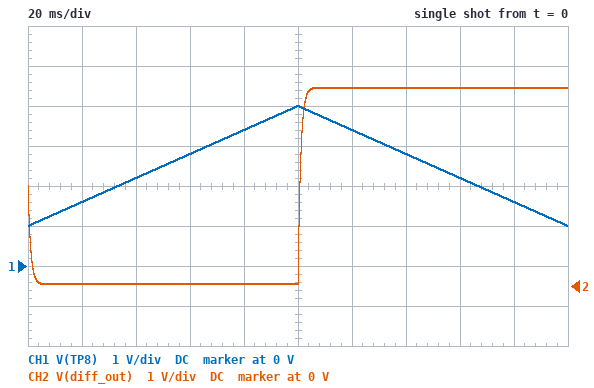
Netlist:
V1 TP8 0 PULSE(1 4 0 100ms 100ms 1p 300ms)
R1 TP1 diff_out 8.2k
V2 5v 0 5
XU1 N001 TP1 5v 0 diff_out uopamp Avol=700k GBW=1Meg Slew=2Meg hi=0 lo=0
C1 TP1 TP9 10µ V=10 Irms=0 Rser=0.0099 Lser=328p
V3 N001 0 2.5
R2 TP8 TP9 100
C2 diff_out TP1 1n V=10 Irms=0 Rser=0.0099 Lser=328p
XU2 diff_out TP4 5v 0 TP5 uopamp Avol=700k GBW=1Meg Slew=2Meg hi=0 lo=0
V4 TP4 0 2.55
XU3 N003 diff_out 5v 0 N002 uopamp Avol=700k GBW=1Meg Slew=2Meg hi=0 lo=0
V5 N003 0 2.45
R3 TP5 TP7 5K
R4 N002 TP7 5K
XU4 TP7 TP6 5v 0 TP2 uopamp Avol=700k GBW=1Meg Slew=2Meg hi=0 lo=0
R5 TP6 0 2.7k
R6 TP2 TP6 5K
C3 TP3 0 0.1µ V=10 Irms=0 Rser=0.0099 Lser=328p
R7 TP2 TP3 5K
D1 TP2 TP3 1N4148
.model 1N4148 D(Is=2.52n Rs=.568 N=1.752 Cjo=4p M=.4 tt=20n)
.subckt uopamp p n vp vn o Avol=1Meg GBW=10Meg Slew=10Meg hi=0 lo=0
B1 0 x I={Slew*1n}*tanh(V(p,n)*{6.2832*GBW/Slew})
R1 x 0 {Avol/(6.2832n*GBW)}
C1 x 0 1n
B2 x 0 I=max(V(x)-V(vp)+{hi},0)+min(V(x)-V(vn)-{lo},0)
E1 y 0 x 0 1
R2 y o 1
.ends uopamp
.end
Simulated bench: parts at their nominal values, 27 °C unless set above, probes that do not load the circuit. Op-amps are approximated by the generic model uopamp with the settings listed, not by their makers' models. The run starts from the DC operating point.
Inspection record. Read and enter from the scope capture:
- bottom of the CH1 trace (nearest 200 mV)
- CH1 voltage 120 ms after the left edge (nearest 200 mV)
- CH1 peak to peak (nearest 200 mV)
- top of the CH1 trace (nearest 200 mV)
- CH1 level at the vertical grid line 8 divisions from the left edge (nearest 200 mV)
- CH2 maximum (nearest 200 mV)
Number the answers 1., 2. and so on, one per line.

1. 1.0 V
2. 3.4 V
3. 3.0 V
4. 4.0 V
5. 2.2 V
6. 5.0 V
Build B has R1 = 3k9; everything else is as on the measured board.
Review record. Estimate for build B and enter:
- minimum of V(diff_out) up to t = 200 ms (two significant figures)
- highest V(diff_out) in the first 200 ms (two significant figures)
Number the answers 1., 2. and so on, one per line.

1. 1.3 V
2. 3.7 V
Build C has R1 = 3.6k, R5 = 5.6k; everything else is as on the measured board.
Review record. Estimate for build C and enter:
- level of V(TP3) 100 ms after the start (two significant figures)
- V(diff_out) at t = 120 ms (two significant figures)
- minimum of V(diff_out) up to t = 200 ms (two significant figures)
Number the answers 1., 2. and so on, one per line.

1. 4.7 V
2. 3.6 V
3. 1.4 V
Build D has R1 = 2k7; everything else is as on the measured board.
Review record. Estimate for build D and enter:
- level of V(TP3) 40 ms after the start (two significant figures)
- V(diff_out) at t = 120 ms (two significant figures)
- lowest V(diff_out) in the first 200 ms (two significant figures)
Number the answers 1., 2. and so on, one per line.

1. 5.0 V
2. 3.3 V
3. 1.7 V
